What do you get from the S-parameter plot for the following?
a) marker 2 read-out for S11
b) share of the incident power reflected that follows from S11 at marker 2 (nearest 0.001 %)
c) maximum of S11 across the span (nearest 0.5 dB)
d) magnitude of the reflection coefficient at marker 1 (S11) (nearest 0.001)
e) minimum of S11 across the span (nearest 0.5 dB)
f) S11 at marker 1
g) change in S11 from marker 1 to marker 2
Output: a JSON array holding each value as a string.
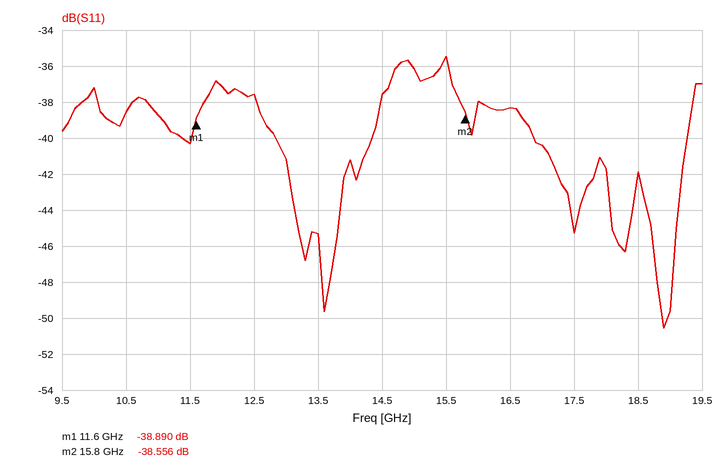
["-38.556 dB", "0.014 %", "-35.5 dB", "0.011", "-50.5 dB", "-38.890 dB", "0.334 dB"]
